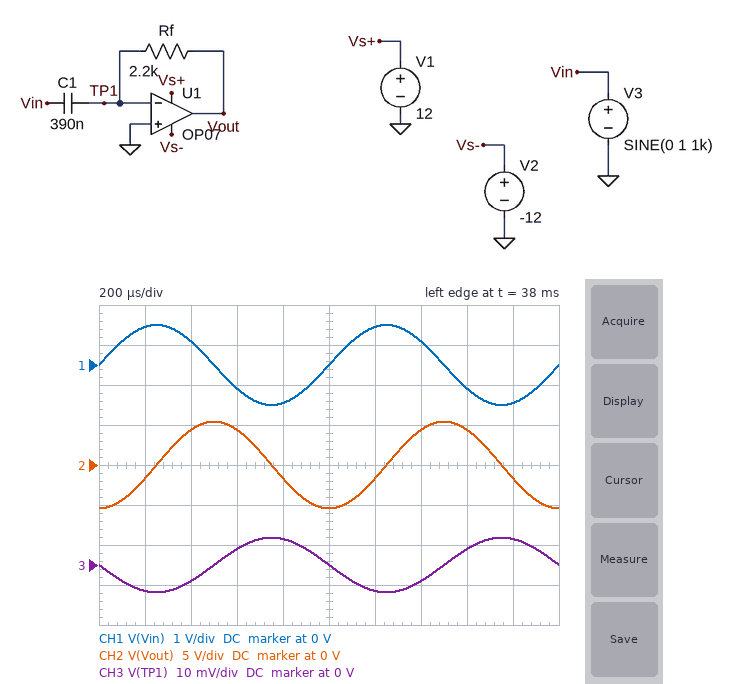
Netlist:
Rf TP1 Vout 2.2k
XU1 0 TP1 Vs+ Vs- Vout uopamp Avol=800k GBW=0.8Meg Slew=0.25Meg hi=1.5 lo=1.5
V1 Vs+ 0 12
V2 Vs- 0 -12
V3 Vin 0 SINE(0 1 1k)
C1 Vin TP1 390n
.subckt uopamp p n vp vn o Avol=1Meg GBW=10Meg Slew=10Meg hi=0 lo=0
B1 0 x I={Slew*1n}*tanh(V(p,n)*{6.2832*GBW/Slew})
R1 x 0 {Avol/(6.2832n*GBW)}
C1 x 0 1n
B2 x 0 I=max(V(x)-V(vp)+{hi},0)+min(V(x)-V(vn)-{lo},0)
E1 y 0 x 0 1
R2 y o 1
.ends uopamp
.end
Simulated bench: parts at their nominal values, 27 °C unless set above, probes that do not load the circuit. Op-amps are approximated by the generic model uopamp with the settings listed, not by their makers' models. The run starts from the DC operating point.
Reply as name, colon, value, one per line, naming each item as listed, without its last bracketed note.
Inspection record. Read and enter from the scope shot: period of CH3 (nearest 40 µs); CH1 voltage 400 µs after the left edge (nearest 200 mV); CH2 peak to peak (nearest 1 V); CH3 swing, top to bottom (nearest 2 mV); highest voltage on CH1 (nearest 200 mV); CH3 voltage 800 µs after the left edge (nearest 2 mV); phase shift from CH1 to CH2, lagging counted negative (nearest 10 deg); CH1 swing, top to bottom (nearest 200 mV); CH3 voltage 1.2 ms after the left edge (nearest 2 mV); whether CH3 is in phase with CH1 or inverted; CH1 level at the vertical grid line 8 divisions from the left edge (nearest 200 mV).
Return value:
period of CH3: 1.00 ms
CH1 voltage 400 µs after the left edge: 600 mV
CH2 peak to peak: 11 V
CH3 swing, top to bottom: 14 mV
highest voltage on CH1: 1.0 V
CH3 voltage 800 µs after the left edge: 6 mV
phase shift from CH1 to CH2, lagging counted negative: -90 deg
CH1 swing, top to bottom: 2.0 V
CH3 voltage 1.2 ms after the left edge: -6 mV
whether CH3 is in phase with CH1 or inverted: inverted
CH1 level at the vertical grid line 8 divisions from the left edge: -600 mV
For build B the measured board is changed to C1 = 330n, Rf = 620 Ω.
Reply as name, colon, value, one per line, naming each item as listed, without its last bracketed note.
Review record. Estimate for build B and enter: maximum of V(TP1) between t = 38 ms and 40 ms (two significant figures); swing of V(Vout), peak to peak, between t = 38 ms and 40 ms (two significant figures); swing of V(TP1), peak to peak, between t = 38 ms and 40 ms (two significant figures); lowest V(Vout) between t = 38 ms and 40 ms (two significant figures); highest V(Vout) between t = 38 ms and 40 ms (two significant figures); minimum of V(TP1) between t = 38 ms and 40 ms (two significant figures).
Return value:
maximum of V(TP1) between t = 38 ms and 40 ms: 1.6 mV
swing of V(Vout), peak to peak, between t = 38 ms and 40 ms: 2.6 V
swing of V(TP1), peak to peak, between t = 38 ms and 40 ms: 3.2 mV
lowest V(Vout) between t = 38 ms and 40 ms: -1.3 V
highest V(Vout) between t = 38 ms and 40 ms: 1.3 V
minimum of V(TP1) between t = 38 ms and 40 ms: -1.6 mV
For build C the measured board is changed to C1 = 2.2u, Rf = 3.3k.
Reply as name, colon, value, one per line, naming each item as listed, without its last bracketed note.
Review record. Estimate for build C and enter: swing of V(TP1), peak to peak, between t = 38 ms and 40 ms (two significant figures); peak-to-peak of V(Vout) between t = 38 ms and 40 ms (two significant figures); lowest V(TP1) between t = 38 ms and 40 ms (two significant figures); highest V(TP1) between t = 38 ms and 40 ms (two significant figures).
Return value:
swing of V(TP1), peak to peak, between t = 38 ms and 40 ms: 2.0 V
peak-to-peak of V(Vout) between t = 38 ms and 40 ms: 21 V
lowest V(TP1) between t = 38 ms and 40 ms: -1.0 V
highest V(TP1) between t = 38 ms and 40 ms: 1.0 V
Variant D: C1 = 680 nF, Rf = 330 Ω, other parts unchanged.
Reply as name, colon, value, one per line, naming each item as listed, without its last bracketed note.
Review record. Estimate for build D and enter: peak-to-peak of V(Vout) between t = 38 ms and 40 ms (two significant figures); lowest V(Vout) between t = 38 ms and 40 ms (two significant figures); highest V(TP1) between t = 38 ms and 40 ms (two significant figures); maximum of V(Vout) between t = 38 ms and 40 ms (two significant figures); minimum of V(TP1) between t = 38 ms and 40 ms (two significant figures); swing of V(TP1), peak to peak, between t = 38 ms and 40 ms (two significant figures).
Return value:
peak-to-peak of V(Vout) between t = 38 ms and 40 ms: 2.8 V
lowest V(Vout) between t = 38 ms and 40 ms: -1.4 V
highest V(TP1) between t = 38 ms and 40 ms: 1.8 mV
maximum of V(Vout) between t = 38 ms and 40 ms: 1.4 V
minimum of V(TP1) between t = 38 ms and 40 ms: -1.8 mV
swing of V(TP1), peak to peak, between t = 38 ms and 40 ms: 3.5 mV
